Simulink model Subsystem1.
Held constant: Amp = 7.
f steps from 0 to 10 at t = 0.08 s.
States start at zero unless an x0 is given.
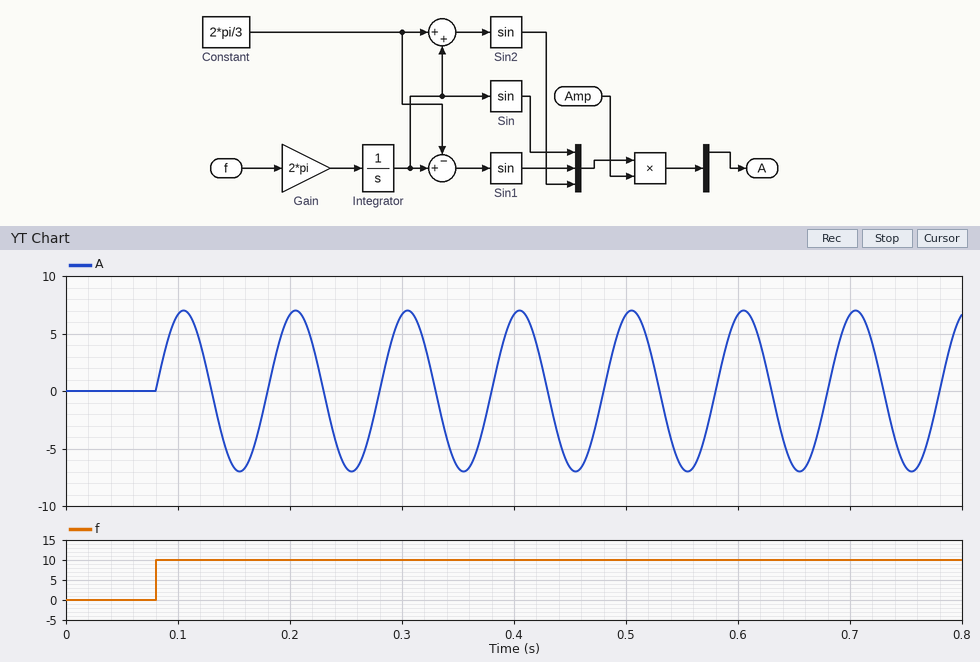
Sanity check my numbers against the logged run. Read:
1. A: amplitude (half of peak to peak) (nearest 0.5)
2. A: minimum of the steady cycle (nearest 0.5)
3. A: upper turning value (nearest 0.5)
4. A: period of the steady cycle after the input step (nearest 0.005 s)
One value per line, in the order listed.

7.0
-7.0
7.0
0.100 s
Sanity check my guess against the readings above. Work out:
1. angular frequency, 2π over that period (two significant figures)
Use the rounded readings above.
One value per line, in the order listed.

63 rad/s
